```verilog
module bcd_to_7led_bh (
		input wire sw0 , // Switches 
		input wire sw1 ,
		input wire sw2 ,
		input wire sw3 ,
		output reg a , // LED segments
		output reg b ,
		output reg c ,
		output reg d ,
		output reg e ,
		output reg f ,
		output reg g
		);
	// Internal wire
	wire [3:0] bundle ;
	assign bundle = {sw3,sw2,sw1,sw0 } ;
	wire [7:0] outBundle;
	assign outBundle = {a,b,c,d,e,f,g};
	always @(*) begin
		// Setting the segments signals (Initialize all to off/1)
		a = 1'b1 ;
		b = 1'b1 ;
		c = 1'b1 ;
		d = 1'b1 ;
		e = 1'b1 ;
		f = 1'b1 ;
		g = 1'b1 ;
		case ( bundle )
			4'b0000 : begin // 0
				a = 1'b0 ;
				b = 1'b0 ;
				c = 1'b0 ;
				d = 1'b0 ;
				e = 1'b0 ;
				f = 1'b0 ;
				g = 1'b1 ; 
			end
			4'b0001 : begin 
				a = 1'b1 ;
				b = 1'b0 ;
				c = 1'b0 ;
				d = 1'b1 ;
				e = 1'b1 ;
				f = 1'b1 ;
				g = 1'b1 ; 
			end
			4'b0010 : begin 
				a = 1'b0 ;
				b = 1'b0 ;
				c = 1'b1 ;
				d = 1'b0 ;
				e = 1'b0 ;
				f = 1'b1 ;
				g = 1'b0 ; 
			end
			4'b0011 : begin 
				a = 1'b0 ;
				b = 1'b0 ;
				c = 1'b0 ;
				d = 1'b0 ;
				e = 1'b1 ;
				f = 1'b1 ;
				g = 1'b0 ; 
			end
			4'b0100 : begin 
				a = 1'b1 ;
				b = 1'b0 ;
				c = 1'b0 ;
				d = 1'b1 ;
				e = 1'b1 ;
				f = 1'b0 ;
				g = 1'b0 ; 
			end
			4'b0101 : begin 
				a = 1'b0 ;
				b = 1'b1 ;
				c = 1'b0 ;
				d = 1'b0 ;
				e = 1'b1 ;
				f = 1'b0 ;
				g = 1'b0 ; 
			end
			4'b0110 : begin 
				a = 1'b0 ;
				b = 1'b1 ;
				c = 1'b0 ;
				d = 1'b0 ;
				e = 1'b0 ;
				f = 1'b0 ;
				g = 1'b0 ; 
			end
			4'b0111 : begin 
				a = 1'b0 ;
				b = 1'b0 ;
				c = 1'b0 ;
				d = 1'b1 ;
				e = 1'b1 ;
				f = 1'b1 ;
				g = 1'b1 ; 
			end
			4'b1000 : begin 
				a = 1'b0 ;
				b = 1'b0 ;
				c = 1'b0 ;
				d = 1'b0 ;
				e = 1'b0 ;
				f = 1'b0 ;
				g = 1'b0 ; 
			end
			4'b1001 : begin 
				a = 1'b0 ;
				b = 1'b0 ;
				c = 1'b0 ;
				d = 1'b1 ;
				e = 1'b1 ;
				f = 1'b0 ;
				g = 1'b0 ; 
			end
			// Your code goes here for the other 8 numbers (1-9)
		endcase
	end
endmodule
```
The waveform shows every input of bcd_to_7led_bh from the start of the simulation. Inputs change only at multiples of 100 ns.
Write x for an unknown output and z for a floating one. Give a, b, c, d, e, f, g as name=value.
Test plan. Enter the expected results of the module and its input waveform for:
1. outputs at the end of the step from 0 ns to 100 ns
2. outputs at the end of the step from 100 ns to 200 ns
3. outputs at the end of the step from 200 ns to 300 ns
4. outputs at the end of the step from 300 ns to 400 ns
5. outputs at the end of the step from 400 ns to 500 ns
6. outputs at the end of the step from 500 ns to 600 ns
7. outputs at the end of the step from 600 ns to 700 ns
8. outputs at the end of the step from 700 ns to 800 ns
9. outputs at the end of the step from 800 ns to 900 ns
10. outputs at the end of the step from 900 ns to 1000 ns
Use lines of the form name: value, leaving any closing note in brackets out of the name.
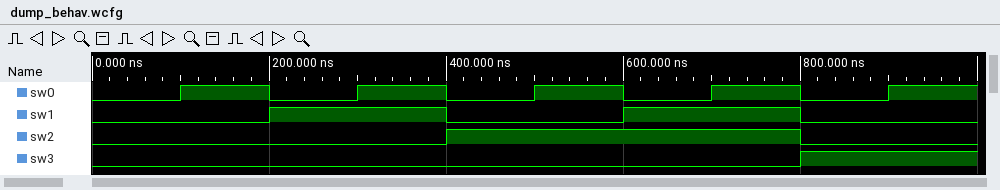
outputs at the end of the step from 0 ns to 100 ns: a=0, b=0, c=0, d=0, e=0, f=0, g=1
outputs at the end of the step from 100 ns to 200 ns: a=1, b=0, c=0, d=1, e=1, f=1, g=1
outputs at the end of the step from 200 ns to 300 ns: a=0, b=0, c=1, d=0, e=0, f=1, g=0
outputs at the end of the step from 300 ns to 400 ns: a=0, b=0, c=0, d=0, e=1, f=1, g=0
outputs at the end of the step from 400 ns to 500 ns: a=1, b=0, c=0, d=1, e=1, f=0, g=0
outputs at the end of the step from 500 ns to 600 ns: a=0, b=1, c=0, d=0, e=1, f=0, g=0
outputs at the end of the step from 600 ns to 700 ns: a=0, b=1, c=0, d=0, e=0, f=0, g=0
outputs at the end of the step from 700 ns to 800 ns: a=0, b=0, c=0, d=1, e=1, f=1, g=1
outputs at the end of the step from 800 ns to 900 ns: a=0, b=0, c=0, d=0, e=0, f=0, g=0
outputs at the end of the step from 900 ns to 1000 ns: a=0, b=0, c=0, d=1, e=1, f=0, g=0
